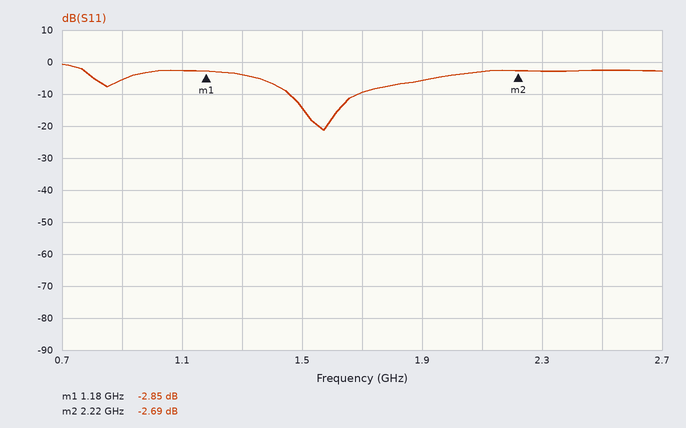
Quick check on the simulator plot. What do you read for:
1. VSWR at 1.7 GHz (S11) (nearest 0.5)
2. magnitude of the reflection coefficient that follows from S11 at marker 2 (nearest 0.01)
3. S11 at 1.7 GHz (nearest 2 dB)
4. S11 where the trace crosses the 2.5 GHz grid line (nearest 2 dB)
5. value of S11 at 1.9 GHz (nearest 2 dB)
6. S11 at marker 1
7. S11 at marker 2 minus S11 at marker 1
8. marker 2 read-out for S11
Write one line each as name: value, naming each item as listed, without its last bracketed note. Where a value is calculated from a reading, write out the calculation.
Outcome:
VSWR at 1.7 GHz (S11): |Γ| = 10^(-10/20) = 0.3162; VSWR = (1 + 0.3162)/(1 − 0.3162) ≈ 1.92, so 2.0 to the nearest 0.5
magnitude of the reflection coefficient that follows from S11 at marker 2: 10^(-2.69/20) ≈ 0.73
S11 at 1.7 GHz: -10 dB
S11 where the trace crosses the 2.5 GHz grid line: -2 dB
value of S11 at 1.9 GHz: -6 dB
S11 at marker 1: -2.85 dB
S11 at marker 2 minus S11 at marker 1: -2.69 − (-2.85) = 0.16 dB
marker 2 read-out for S11: -2.69 dB
